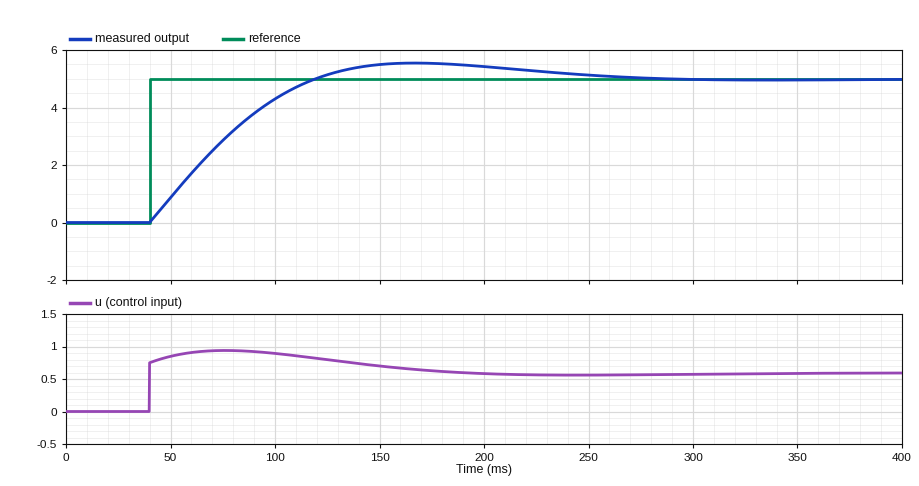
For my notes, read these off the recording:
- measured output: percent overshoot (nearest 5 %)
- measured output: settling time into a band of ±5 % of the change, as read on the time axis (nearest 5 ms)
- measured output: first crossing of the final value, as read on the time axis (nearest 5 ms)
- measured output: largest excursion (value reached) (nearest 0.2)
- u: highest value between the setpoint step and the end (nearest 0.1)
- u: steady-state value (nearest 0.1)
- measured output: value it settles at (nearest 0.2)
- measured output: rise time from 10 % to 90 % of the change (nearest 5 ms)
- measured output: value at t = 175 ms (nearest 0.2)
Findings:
10 %
230 ms
120 ms
5.6
0.9
0.6
5.0
60 ms
5.6
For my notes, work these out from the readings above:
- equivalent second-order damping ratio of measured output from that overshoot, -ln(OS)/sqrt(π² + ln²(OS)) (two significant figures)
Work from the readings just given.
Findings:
0.59
